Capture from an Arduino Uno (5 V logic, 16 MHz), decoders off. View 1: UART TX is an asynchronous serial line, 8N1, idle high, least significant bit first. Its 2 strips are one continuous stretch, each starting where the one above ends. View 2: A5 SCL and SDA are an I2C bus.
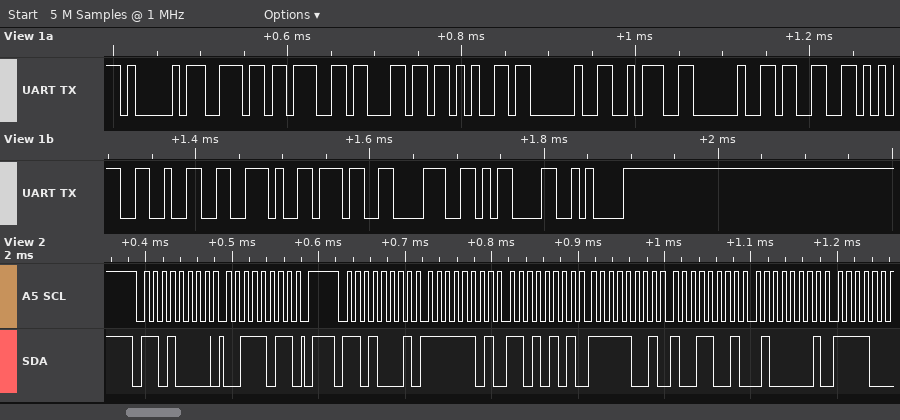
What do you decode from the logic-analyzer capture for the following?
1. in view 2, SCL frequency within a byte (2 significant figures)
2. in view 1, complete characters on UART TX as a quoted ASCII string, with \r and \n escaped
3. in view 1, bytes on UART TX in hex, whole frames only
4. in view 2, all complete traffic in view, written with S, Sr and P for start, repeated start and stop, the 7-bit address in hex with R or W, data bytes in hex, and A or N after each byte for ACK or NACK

100 kHz
"Angle : 352.78\r\n"
41 6E 67 6C 65 20 3A 20 33 35 32 2E 37 38 0D 0A
S 68W A 3B A P S 68R A FD A D5 A F9 A 99 A 41 A
